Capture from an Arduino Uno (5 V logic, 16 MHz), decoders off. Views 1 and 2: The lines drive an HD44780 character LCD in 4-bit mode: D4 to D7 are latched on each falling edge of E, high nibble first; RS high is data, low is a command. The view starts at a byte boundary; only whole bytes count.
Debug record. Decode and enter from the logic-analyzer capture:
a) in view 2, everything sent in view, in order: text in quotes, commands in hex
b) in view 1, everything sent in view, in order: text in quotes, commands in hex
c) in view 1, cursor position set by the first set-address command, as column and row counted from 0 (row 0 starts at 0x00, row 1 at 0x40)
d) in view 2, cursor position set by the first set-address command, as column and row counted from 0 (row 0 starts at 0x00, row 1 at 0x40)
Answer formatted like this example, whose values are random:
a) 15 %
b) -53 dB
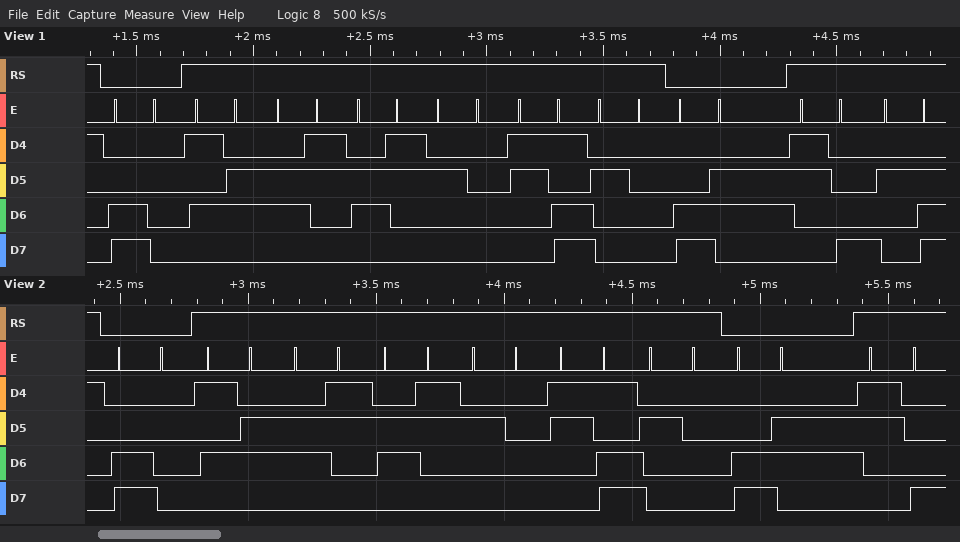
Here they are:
a) 0xC0 "Vcc = " 0xC6 "8"
b) 0xC0 "Vcc = " 0xC6 "8."
c) column 0, row 1
d) column 0, row 1
